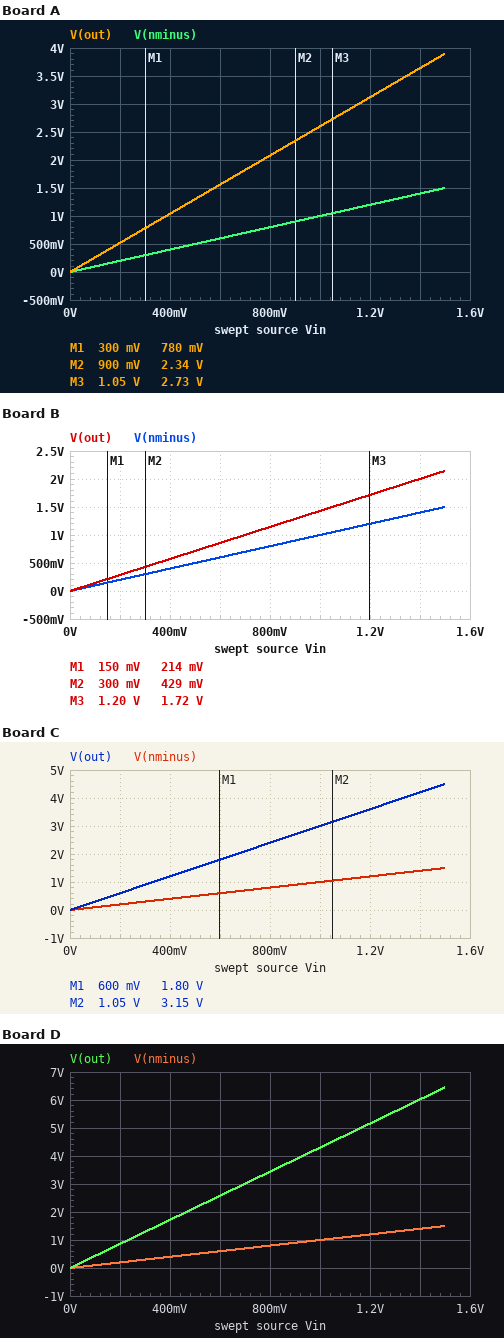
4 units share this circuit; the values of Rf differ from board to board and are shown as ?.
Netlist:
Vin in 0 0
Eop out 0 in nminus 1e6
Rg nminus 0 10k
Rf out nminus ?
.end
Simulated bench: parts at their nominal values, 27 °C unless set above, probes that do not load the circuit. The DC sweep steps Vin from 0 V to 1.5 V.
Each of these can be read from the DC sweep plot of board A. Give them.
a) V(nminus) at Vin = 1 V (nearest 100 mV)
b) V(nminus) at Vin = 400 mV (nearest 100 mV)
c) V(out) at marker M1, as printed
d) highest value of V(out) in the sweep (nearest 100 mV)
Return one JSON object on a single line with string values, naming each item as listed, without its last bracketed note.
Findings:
{"V(nminus) at Vin = 1 V": "1.0 V", "V(nminus) at Vin = 400 mV": "400 mV", "V(out) at marker M1, as printed": "780 mV", "highest value of V(out) in the sweep": "3.9 V"}
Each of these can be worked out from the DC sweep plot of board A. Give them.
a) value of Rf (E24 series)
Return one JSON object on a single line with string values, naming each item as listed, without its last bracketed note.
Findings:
{"value of Rf": "16 kΩ"}
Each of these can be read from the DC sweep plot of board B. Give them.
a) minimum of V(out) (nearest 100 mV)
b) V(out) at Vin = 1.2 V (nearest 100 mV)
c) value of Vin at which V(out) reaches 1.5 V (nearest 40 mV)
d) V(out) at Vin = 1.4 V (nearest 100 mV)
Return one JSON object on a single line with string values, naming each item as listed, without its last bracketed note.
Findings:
{"minimum of V(out)": "0 V", "V(out) at Vin = 1.2 V": "1.7 V", "value of Vin at which V(out) reaches 1.5 V": "1.04 V", "V(out) at Vin = 1.4 V": "2.0 V"}
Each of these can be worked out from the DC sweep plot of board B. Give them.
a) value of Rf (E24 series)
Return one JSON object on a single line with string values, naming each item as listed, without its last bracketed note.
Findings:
{"value of Rf": "4.3 kΩ"}
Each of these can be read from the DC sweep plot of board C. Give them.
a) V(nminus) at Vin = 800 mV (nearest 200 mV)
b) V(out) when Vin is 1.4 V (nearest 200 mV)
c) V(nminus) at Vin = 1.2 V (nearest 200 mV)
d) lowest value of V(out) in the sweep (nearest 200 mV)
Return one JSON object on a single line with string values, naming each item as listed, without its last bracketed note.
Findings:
{"V(nminus) at Vin = 800 mV": "800 mV", "V(out) when Vin is 1.4 V": "4.2 V", "V(nminus) at Vin = 1.2 V": "1.2 V", "lowest value of V(out) in the sweep": "0 V"}
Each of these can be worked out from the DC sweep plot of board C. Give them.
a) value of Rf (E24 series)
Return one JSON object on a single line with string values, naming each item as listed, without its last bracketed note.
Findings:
{"value of Rf": "20 kΩ"}
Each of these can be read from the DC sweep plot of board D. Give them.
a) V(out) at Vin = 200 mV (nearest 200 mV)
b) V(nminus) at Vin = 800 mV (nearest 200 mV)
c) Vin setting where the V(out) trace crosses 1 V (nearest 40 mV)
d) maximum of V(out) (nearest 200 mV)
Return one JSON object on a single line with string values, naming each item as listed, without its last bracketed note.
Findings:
{"V(out) at Vin = 200 mV": "800 mV", "V(nminus) at Vin = 800 mV": "800 mV", "Vin setting where the V(out) trace crosses 1 V": "240 mV", "maximum of V(out)": "6.4 V"}
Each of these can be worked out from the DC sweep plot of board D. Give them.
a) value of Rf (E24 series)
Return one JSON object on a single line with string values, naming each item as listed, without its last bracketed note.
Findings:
{"value of Rf": "33 kΩ"}
